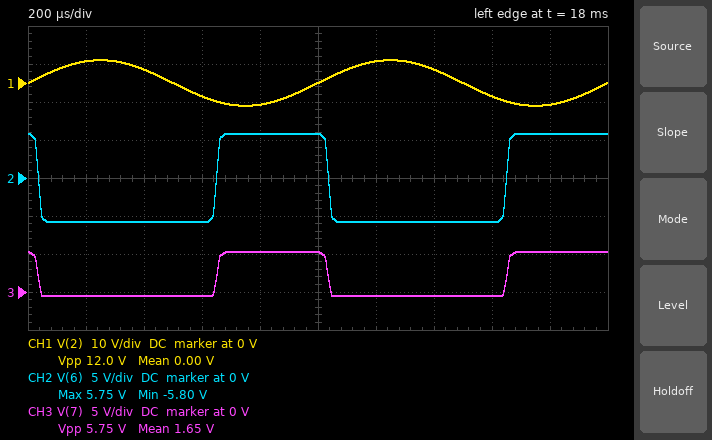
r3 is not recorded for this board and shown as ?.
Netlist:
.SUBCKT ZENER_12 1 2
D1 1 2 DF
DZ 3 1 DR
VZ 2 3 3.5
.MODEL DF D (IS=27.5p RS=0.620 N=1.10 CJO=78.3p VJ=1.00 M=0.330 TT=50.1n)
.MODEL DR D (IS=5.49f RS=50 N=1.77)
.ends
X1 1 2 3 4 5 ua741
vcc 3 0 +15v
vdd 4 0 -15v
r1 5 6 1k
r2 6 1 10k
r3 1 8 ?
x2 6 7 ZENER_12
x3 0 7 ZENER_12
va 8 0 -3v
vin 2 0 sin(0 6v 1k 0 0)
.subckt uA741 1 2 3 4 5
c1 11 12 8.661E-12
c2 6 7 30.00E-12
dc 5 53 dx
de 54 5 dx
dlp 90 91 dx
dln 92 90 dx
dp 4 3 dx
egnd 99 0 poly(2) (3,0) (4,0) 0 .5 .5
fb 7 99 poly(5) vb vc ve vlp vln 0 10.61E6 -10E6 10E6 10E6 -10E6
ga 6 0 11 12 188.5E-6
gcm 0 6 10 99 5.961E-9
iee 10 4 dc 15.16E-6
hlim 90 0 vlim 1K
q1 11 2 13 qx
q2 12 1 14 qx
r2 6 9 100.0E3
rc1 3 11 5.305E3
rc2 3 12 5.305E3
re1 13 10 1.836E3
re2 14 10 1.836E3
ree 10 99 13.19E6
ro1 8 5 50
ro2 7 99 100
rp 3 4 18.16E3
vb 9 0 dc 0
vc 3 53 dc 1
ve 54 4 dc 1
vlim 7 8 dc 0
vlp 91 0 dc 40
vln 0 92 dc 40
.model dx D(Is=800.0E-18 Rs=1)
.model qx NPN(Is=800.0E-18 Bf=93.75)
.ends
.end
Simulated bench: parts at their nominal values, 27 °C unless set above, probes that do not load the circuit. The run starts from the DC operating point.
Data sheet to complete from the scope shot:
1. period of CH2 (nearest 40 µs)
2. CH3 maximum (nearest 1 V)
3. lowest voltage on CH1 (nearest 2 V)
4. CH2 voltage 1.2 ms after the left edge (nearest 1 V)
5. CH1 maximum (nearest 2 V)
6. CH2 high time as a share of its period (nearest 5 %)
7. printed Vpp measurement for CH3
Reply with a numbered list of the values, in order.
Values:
1. 1.00 ms
2. 5 V
3. -6 V
4. -6 V
5. 6 V
6. 40 %
7. 5.75 V
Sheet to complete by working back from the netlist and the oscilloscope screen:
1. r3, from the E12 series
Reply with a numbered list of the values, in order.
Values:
1. 5.6 kΩ
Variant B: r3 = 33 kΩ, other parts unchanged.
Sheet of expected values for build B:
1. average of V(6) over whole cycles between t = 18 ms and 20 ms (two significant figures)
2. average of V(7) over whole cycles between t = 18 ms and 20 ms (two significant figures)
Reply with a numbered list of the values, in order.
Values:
1. -680 mV
2. 2.0 V
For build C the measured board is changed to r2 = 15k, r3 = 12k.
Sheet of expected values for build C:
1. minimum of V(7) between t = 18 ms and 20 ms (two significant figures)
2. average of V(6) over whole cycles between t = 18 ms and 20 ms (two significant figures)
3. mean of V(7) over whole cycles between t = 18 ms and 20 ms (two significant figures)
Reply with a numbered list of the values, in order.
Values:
1. -560 mV
2. -1.2 V
3. 1.7 V
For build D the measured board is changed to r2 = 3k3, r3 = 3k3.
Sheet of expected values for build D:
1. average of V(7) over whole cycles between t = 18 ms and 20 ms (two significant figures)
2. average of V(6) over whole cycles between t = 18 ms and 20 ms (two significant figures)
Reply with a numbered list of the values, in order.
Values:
1. 1.7 V
2. -1.1 V
